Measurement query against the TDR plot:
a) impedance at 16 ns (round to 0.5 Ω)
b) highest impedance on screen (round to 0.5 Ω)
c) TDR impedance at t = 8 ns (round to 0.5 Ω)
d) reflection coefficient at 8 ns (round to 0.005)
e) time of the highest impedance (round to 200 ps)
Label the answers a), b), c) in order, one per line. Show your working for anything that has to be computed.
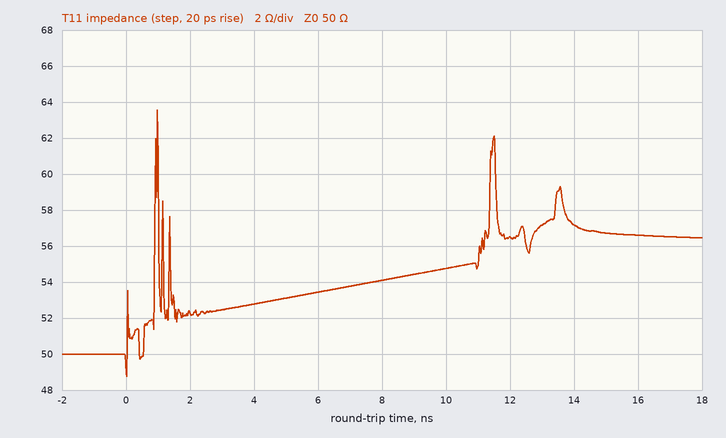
a) 56.5 Ω
b) 63.5 Ω
c) 54.0 Ω
d) (54 − 50)/(54 + 50) ≈ +0.0385, so +0.040 to the nearest 0.005
e) 1.0 ns
